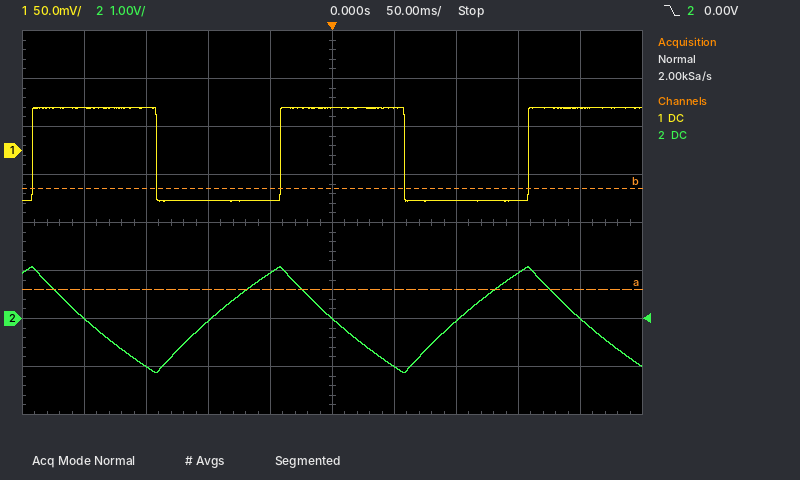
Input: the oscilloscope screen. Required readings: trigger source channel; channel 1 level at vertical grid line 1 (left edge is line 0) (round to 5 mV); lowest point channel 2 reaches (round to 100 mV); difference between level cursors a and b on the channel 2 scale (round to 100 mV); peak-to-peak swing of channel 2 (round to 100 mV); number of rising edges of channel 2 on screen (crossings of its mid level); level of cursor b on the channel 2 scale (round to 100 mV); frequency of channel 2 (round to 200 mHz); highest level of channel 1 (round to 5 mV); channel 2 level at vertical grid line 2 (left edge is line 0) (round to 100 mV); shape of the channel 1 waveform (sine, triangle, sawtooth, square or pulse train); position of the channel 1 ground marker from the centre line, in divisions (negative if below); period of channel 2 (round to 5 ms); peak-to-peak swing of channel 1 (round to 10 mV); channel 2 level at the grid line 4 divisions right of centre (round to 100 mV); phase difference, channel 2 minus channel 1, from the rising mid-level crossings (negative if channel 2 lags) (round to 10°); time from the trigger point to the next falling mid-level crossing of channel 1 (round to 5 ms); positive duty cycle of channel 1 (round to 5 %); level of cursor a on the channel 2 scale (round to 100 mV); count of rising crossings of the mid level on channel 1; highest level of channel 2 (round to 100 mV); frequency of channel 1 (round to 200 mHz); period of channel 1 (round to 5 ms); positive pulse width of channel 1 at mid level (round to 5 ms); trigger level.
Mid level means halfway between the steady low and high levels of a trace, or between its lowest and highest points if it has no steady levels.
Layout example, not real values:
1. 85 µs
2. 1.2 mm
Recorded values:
1. channel 2
2. 45 mV
3. -1.1 V
4. 2.1 V
5. 2.2 V
6. 2
7. 2.7 V
8. 5.0 Hz
9. 45 mV
10. -1.0 V
11. square
12. +1.5 div
13. 200 ms
14. 100 mV
15. 0.0 V
16. +100°
17. 60 ms
18. 50 %
19. 600 mV
20. 3
21. 1.1 V
22. 5.0 Hz
23. 200 ms
24. 100 ms
25. 0.00 V
